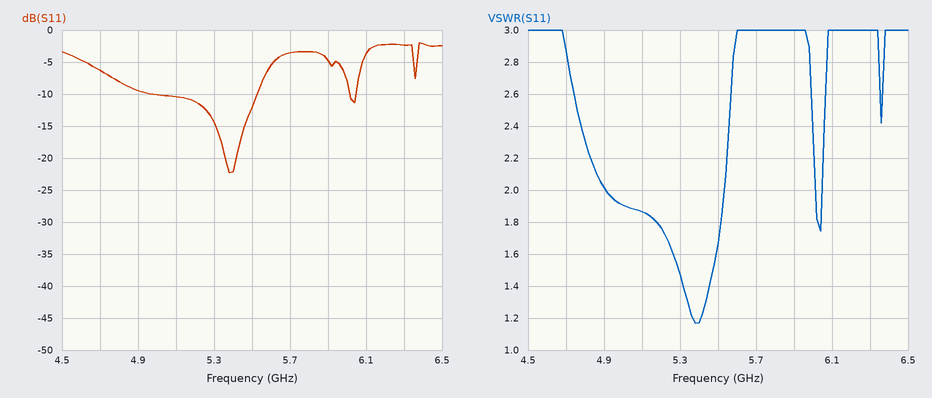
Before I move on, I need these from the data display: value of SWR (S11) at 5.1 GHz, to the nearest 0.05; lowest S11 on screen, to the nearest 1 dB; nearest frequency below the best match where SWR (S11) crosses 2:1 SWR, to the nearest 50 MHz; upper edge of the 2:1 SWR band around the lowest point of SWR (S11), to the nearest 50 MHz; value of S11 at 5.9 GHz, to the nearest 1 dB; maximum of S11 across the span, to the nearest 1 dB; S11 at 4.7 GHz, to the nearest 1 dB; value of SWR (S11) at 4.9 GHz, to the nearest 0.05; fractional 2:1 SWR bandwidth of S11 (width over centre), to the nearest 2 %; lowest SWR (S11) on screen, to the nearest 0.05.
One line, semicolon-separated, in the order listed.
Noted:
1.85; -22 dB; 4.90 GHz; 5.55 GHz; -5 dB; -2 dB; -6 dB; 2.00; 12 %; 1.15
